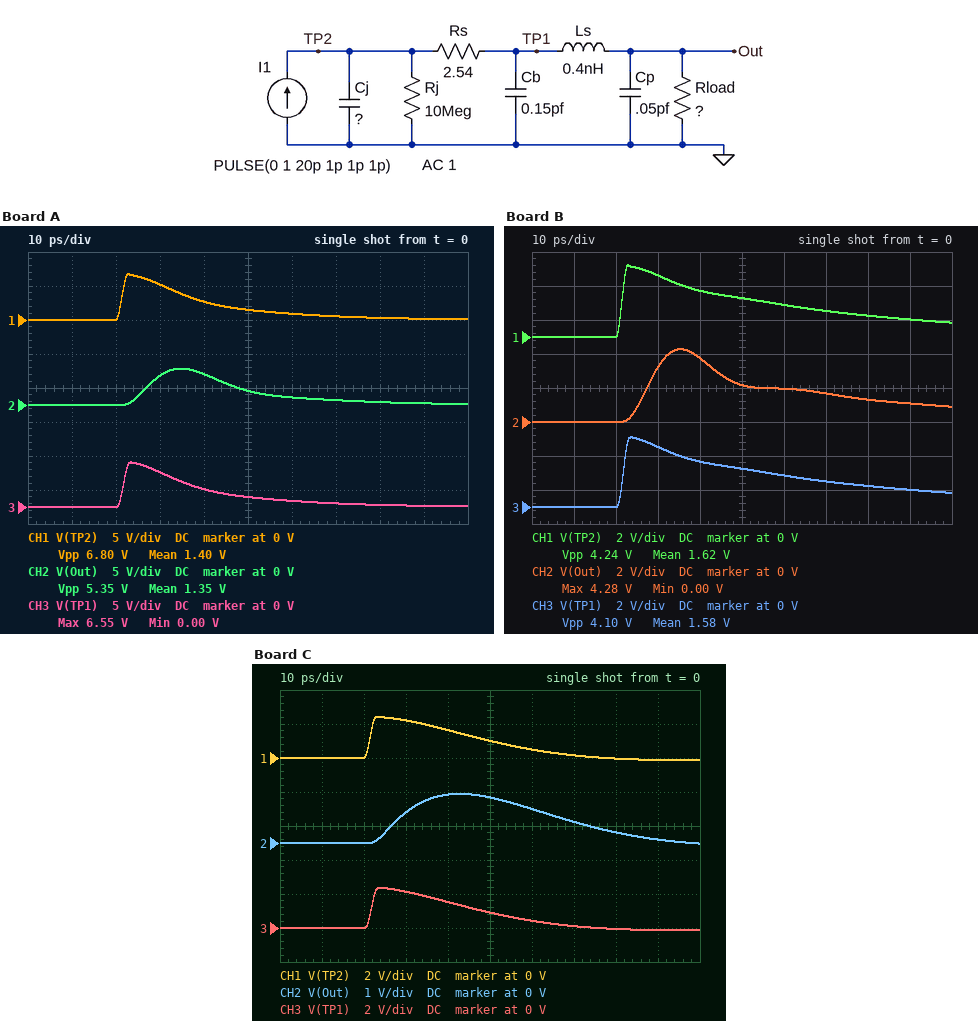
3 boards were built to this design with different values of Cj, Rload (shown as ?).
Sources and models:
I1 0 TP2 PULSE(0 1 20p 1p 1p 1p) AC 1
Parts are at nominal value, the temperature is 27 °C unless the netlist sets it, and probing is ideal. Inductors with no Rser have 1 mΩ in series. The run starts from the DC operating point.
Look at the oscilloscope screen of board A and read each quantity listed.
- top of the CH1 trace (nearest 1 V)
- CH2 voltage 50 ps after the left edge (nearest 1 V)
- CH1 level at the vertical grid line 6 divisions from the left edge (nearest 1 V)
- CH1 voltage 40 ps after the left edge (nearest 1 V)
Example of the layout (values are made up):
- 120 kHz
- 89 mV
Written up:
- 7 V
- 2 V
- 1 V
- 3 V
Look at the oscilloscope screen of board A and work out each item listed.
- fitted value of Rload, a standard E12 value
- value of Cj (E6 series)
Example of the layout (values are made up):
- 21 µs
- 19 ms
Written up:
- 68 Ω
- 150 fF
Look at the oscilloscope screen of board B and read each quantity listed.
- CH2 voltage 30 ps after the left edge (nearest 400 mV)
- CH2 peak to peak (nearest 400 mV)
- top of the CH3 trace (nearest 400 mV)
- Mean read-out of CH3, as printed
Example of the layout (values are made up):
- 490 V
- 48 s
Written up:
- 3.2 V
- 4.4 V
- 4.0 V
- 1.58 V
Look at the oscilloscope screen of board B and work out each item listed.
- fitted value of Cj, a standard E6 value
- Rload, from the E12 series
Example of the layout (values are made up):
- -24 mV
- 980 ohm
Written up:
- 330 fF
- 100 Ω
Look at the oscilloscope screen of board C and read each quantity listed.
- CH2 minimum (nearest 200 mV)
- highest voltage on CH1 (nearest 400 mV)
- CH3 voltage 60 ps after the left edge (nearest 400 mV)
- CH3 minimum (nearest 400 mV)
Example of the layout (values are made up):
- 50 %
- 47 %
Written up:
- 0 V
- 2.4 V
- 400 mV
- 0 V
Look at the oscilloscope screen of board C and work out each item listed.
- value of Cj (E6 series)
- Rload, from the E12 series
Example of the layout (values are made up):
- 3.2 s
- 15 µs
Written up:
- 680 fF
- 27 Ω
